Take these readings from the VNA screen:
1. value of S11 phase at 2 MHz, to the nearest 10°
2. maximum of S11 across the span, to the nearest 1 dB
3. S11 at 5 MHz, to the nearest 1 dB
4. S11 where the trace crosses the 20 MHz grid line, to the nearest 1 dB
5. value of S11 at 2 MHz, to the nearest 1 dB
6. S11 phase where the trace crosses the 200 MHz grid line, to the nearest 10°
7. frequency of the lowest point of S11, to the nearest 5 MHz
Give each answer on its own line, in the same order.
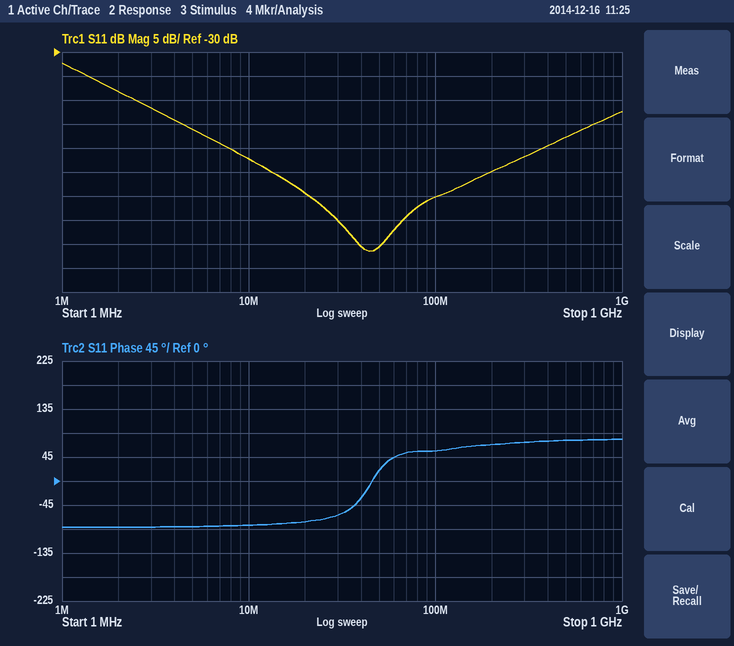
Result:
-90°
-32 dB
-46 dB
-59 dB
-38 dB
70°
45 MHz
